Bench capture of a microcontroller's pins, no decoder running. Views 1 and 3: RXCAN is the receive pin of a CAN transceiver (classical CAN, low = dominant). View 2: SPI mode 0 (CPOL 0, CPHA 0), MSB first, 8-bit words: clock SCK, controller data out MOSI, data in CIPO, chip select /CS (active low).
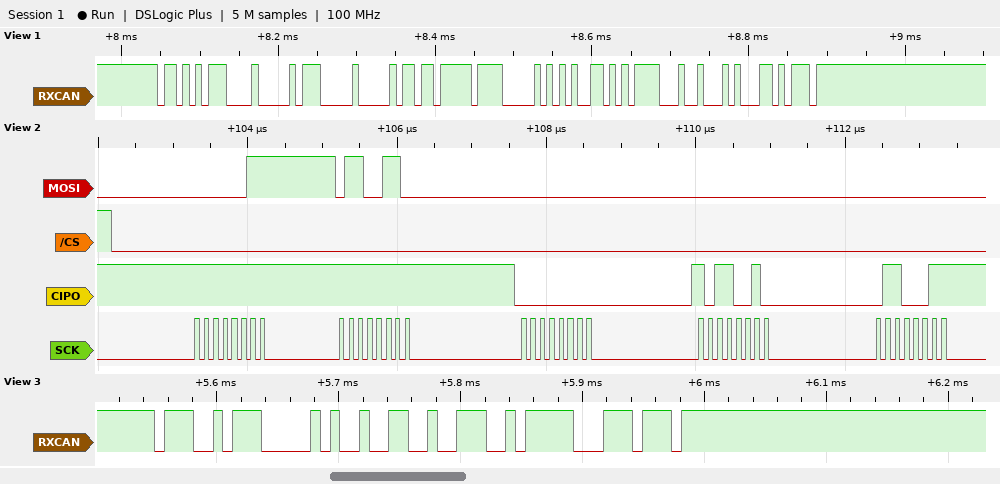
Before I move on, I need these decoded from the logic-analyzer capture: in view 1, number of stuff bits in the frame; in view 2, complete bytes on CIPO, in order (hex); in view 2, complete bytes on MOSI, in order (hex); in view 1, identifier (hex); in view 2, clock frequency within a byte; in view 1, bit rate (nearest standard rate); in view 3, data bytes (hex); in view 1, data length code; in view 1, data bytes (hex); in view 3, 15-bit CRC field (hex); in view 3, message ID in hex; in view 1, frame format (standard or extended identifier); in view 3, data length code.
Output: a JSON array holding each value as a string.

["5", "FF FF 00 B2 63", "03 66 00 00 00", "0x6AE", "8 MHz", "125 kbit/s", "4C 9C", "8", "1C 00 6D FF 02 A6 AF 12", "0x5F3B", "0x72E", "standard", "2"]
